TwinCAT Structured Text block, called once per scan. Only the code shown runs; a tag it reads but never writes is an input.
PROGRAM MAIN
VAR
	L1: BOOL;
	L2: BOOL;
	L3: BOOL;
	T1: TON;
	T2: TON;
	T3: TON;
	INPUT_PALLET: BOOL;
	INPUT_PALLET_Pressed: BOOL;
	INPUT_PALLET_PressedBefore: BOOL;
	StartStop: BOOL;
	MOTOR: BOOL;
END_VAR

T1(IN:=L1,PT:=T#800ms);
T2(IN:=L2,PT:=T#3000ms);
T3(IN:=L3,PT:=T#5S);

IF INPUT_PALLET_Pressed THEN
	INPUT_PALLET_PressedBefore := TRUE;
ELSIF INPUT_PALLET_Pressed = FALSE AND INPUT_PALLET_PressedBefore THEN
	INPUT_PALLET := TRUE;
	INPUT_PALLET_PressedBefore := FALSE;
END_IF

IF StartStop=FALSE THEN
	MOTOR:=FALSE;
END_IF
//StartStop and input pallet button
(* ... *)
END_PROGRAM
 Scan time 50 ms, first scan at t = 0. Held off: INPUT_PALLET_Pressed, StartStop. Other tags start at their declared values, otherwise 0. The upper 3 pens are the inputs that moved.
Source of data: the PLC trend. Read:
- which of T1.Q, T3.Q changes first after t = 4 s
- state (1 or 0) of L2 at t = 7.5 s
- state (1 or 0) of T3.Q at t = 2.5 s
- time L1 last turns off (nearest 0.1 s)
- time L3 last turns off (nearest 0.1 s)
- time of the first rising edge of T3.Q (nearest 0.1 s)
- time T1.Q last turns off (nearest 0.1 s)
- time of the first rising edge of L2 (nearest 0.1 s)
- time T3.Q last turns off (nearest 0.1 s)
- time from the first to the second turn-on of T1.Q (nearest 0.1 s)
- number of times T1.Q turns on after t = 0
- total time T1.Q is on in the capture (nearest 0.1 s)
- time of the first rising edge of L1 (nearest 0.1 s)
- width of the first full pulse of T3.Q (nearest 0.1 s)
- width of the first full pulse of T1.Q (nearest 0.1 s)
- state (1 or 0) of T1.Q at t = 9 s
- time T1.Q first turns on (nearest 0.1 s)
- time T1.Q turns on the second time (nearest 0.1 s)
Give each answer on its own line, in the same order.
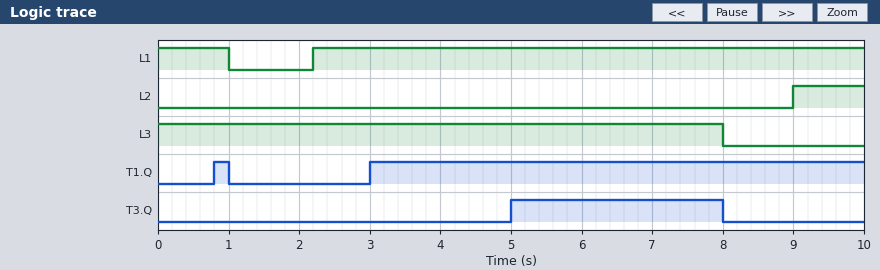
T3.Q
0
0
1.0 s
8.0 s
5.0 s
1.0 s
9.0 s
8.0 s
2.2 s
2
7.2 s
2.2 s
3.0 s
0.2 s
1
0.8 s
3.0 s
